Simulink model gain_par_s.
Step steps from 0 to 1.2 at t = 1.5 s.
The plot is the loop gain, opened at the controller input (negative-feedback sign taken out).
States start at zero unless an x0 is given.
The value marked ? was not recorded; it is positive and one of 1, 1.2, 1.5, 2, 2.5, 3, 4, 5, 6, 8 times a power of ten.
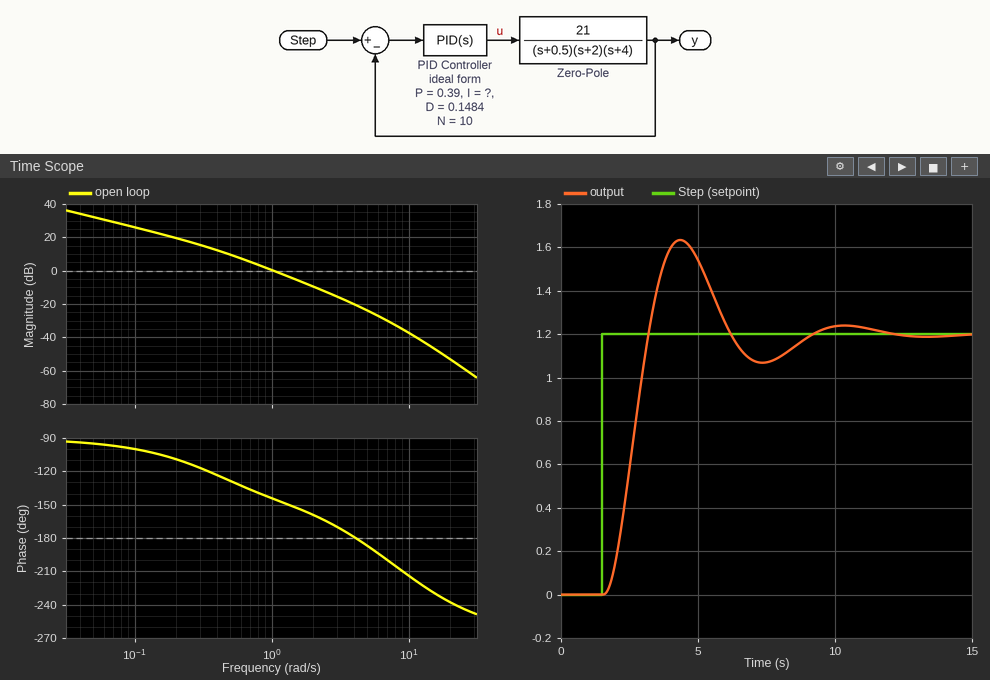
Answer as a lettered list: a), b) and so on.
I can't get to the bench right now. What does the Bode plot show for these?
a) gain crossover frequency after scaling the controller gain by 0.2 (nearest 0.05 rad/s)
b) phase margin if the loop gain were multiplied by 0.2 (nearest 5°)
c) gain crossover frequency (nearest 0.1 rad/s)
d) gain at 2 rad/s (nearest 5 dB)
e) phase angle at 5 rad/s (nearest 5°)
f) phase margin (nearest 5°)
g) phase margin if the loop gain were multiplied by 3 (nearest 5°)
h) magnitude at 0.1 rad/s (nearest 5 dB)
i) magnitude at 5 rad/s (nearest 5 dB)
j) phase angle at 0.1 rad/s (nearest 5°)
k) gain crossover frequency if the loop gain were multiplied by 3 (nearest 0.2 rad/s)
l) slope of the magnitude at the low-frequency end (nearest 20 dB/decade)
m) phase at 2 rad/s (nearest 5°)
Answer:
a) 0.35 rad/s
b) 60°
c) 1.0 rad/s
d) -10 dB
e) -185°
f) 35°
g) 20°
h) 25 dB
i) -25 dB
j) -100°
k) 2.0 rad/s
l) -20 dB/decade
m) -160°
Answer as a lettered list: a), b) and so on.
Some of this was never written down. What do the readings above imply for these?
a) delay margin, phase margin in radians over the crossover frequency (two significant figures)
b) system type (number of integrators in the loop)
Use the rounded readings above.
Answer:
a) 0.61 s
b) 1
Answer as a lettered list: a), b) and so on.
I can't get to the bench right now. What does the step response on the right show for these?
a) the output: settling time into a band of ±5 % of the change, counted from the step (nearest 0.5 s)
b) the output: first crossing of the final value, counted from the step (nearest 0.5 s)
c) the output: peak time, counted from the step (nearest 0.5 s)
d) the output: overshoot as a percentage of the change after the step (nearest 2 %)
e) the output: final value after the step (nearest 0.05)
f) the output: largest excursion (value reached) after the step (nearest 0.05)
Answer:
a) 7.0 s
b) 1.5 s
c) 3.0 s
d) 36 %
e) 1.20
f) 1.65
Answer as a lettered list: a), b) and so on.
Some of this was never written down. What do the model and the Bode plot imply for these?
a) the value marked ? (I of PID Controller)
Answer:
a) 1
